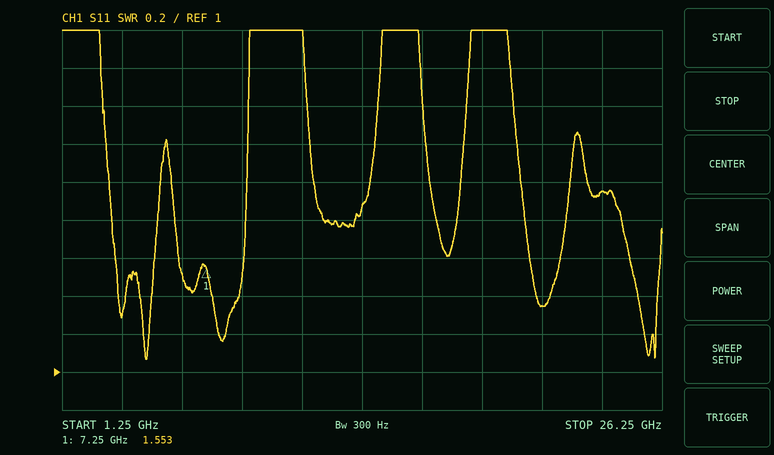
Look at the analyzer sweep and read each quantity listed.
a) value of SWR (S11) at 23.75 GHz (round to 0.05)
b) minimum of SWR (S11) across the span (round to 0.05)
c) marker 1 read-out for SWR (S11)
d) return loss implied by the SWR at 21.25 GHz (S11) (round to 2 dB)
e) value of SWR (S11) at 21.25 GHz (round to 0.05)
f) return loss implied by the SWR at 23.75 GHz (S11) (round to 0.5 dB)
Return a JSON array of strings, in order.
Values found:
["1.95", "1.05", "1.553", "16 dB", "1.35", "10.0 dB"]
